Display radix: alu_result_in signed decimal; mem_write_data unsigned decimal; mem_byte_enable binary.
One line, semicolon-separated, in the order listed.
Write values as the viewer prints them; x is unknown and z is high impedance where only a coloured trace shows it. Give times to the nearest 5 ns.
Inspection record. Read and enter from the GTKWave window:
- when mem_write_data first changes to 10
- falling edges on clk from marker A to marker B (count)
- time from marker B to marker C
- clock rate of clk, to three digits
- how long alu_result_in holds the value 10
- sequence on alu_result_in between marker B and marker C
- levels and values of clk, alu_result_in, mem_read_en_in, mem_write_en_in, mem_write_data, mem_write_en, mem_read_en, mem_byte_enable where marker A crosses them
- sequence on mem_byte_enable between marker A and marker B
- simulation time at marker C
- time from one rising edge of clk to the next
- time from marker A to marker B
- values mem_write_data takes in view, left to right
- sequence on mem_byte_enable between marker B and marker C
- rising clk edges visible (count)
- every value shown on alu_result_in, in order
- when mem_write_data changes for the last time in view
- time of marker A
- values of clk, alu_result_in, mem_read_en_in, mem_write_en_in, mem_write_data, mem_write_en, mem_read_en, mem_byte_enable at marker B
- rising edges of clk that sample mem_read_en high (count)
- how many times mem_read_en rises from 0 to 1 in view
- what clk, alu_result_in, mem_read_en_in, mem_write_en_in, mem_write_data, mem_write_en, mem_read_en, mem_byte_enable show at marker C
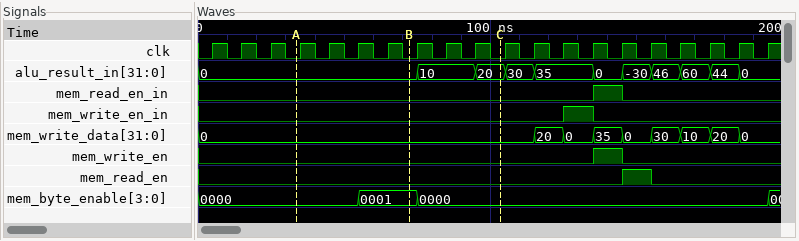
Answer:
165 ns; 4; 30 ns; 100 MHz; 20 ns; 0, 10, 20; clk=0, alu_result_in=0, mem_read_en_in=0, mem_write_en_in=0, mem_write_data=0, mem_write_en=0, mem_read_en=0, mem_byte_enable=0000; 0000, 0001; 105 ns; 10 ns; 40 ns; 0, 20, 0, 35, 0, 30, 10, 20, 0; 0001, 0000; 20; 0, 10, 20, 30, 35, 0, -30, 46, 60, 44, 0; 185 ns; 35 ns; clk=0, alu_result_in=0, mem_read_en_in=0, mem_write_en_in=0, mem_write_data=0, mem_write_en=0, mem_read_en=0, mem_byte_enable=0001; 1; 1; clk=0, alu_result_in=20, mem_read_en_in=0, mem_write_en_in=0, mem_write_data=0, mem_write_en=0, mem_read_en=0, mem_byte_enable=0000
